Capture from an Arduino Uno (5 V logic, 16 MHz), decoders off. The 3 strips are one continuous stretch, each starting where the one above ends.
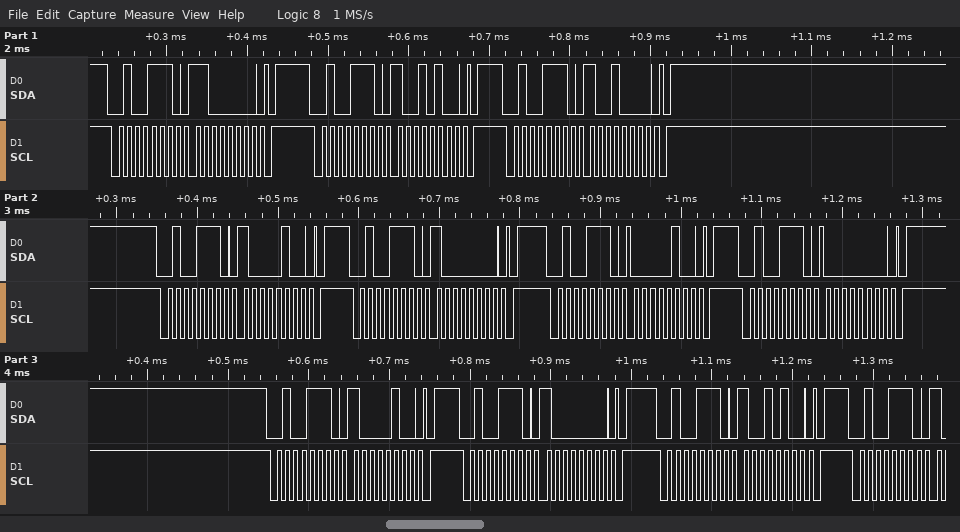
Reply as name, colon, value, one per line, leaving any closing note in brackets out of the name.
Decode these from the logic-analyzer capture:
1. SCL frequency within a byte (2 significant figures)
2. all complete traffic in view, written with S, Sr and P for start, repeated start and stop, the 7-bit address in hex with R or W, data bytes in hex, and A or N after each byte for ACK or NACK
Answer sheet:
SCL frequency within a byte: 100 kHz
all complete traffic in view, written with S, Sr and P for start, repeated start and stop, the 7-bit address in hex with R or W, data bytes in hex, and A or N after each byte for ACK or NACK: S 27W A C0 A P S 27W A 94 A P S 27W A 90 A P S 27W A 84 A P S 27W A 80 A P S 27W A 04 A P S 27W A 00 A P S 27W A 84 A P S 27W A 80 A P S 27W A 94 A P S 27W A
